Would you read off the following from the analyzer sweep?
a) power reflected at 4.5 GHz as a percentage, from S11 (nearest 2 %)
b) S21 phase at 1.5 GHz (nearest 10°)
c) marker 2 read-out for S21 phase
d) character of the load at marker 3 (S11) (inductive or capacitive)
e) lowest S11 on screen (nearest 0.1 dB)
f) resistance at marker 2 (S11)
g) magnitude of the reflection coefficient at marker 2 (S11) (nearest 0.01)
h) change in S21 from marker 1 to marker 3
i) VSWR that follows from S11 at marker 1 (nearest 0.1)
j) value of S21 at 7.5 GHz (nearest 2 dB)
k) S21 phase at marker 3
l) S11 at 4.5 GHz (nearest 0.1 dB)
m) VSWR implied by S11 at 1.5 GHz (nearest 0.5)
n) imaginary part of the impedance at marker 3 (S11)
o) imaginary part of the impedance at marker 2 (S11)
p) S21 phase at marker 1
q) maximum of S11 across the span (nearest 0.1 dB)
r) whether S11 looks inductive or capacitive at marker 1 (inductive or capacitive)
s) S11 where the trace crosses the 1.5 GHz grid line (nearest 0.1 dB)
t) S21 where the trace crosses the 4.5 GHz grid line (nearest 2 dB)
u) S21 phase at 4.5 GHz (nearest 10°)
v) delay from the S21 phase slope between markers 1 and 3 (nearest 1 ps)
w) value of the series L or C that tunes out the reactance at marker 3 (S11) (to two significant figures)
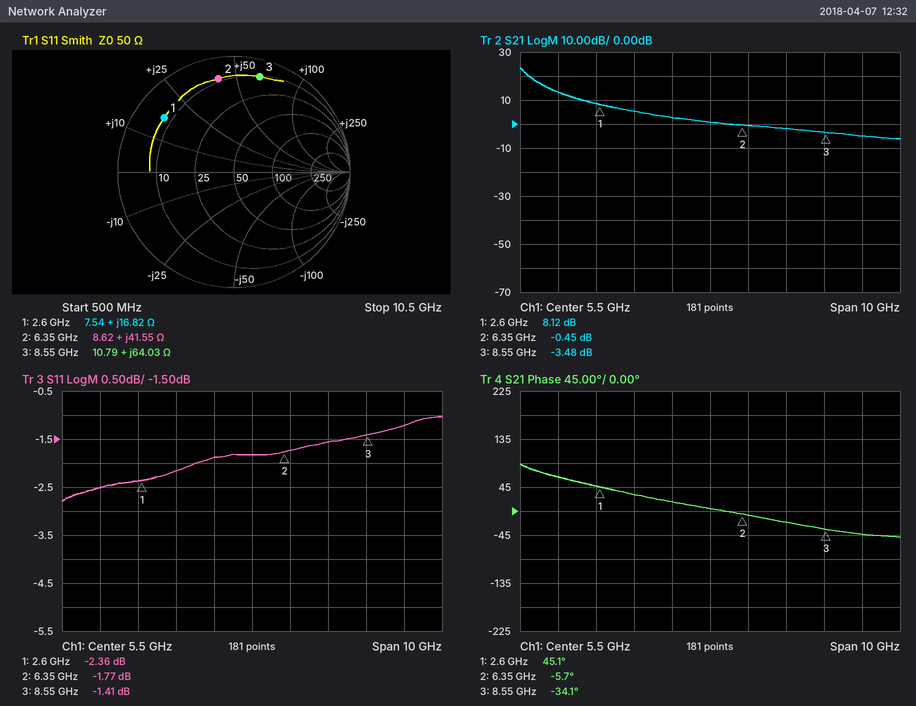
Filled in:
64 %
60°
-5.7°
inductive
-2.8 dB
8.62 Ω
0.82
-11.60 dB
7.4
-2 dB
-34.1°
-1.9 dB
7.0
+64.03 Ω
+41.55 Ω
45.1°
-1.0 dB
inductive
-2.5 dB
2 dB
20°
37 ps
290 fF
